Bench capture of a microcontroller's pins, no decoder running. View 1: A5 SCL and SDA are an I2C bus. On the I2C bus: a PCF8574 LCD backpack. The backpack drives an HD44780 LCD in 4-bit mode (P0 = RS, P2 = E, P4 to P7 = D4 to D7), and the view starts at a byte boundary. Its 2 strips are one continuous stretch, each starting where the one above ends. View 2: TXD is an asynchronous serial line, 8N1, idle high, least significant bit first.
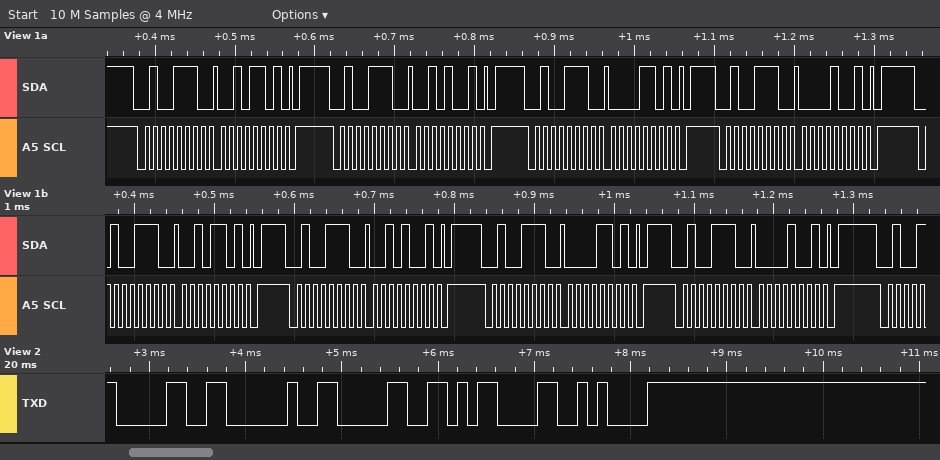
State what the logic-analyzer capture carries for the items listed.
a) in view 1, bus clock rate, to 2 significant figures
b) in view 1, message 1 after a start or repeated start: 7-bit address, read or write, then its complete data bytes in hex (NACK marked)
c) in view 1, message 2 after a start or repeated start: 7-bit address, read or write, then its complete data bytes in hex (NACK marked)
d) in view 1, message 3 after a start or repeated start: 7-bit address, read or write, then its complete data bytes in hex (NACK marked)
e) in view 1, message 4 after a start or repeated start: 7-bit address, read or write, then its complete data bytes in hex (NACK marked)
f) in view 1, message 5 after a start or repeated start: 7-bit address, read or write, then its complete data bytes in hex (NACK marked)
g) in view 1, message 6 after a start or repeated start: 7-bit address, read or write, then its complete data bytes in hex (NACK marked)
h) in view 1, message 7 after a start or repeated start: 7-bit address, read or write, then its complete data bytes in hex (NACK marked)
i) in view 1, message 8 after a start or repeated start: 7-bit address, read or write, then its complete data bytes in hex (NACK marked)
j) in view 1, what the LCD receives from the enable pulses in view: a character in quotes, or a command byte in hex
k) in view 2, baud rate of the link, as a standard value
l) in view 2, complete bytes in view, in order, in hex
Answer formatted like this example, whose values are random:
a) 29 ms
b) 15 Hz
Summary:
a) 100 kHz
b) 0x27 write: 2D
c) 0x27 write: 29
d) 0x27 write: 0D
e) 0x27 write: 09
f) 0x27 write: 2D
g) 0x27 write: 29
h) 0x27 write: 0D
i) 0x27 write: 09
j) ' ' ' '
k) 9600 baud
l) 0x30 0x20 0x30 0x0D 0x0A
